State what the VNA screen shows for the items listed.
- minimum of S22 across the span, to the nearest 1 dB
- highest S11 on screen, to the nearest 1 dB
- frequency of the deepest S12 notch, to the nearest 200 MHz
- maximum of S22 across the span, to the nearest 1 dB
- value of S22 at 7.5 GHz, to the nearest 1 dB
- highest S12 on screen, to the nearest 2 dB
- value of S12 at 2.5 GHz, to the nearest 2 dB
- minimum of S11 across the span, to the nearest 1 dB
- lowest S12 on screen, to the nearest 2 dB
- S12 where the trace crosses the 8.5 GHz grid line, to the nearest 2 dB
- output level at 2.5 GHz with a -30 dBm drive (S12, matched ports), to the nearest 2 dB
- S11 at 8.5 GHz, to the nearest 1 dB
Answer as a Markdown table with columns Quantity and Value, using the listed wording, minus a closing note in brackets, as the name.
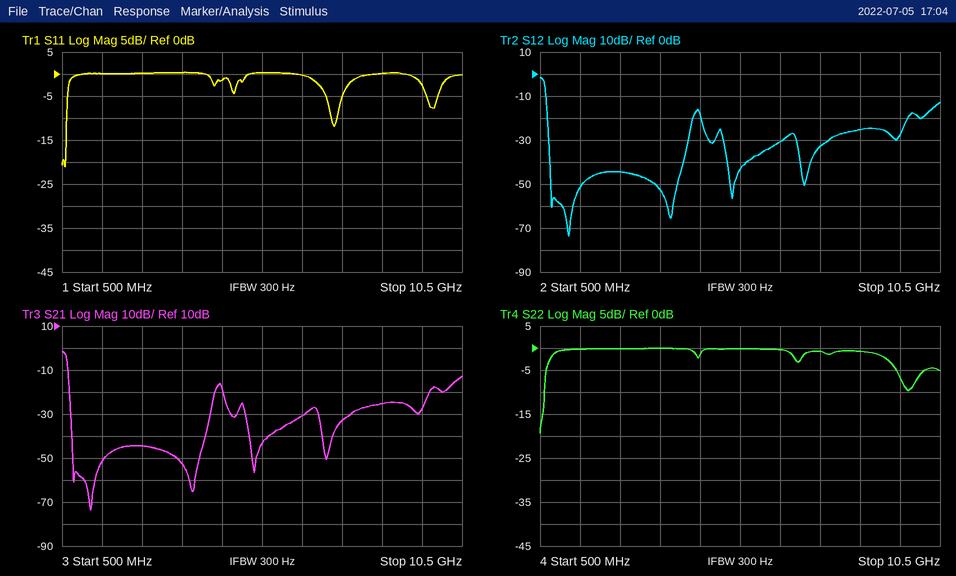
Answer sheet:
| Quantity | Value |
|---|---|
| minimum of S22 across the span, to the nearest 1 dB | -19 dB |
| highest S11 on screen, to the nearest 1 dB | 0 dB |
| frequency of the deepest S12 notch, to the nearest 200 MHz | 1.2 GHz |
| maximum of S22 across the span, to the nearest 1 dB | 0 dB |
| value of S22 at 7.5 GHz, to the nearest 1 dB | -1 dB |
| highest S12 on screen, to the nearest 2 dB | -2 dB |
| value of S12 at 2.5 GHz, to the nearest 2 dB | -44 dB |
| minimum of S11 across the span, to the nearest 1 dB | -21 dB |
| lowest S12 on screen, to the nearest 2 dB | -74 dB |
| S12 where the trace crosses the 8.5 GHz grid line, to the nearest 2 dB | -26 dB |
| output level at 2.5 GHz with a -30 dBm drive (S12, matched ports), to the nearest 2 dB | -74 dBm |
| S11 at 8.5 GHz, to the nearest 1 dB | 0 dB |
